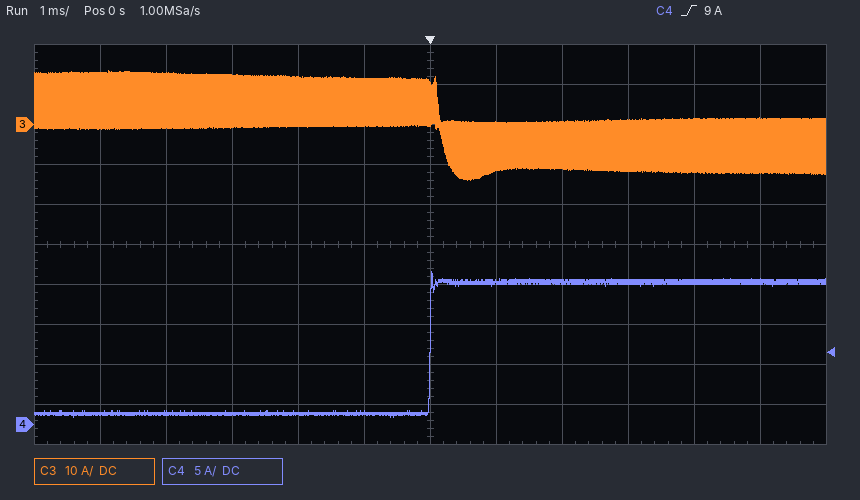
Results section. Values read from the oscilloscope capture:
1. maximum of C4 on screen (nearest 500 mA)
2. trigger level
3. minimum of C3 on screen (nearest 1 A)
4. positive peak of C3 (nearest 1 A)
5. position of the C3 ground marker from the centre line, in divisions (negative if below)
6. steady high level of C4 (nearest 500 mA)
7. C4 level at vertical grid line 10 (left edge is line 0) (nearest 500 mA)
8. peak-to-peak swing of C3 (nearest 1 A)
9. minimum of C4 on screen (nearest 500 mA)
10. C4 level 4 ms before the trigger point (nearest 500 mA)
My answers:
19.0 A
9 A
-14 A
13 A
+3.0 div
18.0 A
18.0 A
27 A
1.0 A
1.5 A
